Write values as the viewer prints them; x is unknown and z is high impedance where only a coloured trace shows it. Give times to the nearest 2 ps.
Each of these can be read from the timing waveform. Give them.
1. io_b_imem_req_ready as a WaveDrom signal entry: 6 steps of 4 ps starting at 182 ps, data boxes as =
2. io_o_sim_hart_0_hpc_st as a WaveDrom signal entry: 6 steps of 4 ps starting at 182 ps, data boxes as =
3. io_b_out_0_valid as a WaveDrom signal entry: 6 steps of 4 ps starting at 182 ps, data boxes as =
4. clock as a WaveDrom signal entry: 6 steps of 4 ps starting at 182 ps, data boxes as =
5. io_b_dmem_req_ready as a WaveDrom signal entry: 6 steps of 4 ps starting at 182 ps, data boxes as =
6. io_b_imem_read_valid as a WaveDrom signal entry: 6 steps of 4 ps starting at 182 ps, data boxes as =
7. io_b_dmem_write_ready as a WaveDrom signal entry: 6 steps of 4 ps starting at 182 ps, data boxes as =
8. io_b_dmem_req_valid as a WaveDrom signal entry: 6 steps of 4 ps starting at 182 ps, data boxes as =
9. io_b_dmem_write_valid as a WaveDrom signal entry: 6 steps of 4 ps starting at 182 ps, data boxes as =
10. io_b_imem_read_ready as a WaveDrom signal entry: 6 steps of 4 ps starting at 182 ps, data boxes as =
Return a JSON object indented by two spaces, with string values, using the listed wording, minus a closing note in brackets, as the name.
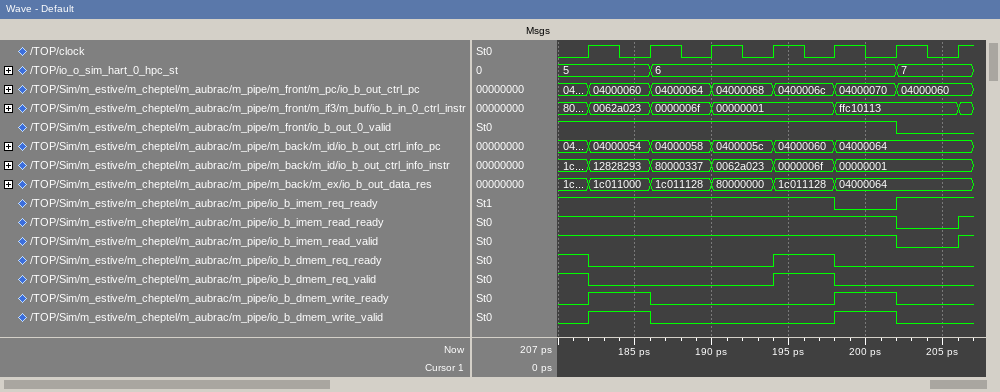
{
  "io_b_imem_req_ready as a WaveDrom signal entry: 6 steps of 4 ps starting at 182 ps, data boxes as =": "{name: 'io_b_imem_req_ready', wave: '1...01'}",
  "io_o_sim_hart_0_hpc_st as a WaveDrom signal entry: 6 steps of 4 ps starting at 182 ps, data boxes as =": "{name: 'io_o_sim_hart_0_hpc_st', wave: '==...=', data: '5 6 7'}",
  "io_b_out_0_valid as a WaveDrom signal entry: 6 steps of 4 ps starting at 182 ps, data boxes as =": "{name: 'io_b_out_0_valid', wave: '1....0'}",
  "clock as a WaveDrom signal entry: 6 steps of 4 ps starting at 182 ps, data boxes as =": "{name: 'clock', wave: 'p.....'}",
  "io_b_dmem_req_ready as a WaveDrom signal entry: 6 steps of 4 ps starting at 182 ps, data boxes as =": "{name: 'io_b_dmem_req_ready', wave: '0..10.'}",
  "io_b_imem_read_valid as a WaveDrom signal entry: 6 steps of 4 ps starting at 182 ps, data boxes as =": "{name: 'io_b_imem_read_valid', wave: '1....0'}",
  "io_b_dmem_write_ready as a WaveDrom signal entry: 6 steps of 4 ps starting at 182 ps, data boxes as =": "{name: 'io_b_dmem_write_ready', wave: '10..10'}",
  "io_b_dmem_req_valid as a WaveDrom signal entry: 6 steps of 4 ps starting at 182 ps, data boxes as =": "{name: 'io_b_dmem_req_valid', wave: '0..10.'}",
  "io_b_dmem_write_valid as a WaveDrom signal entry: 6 steps of 4 ps starting at 182 ps, data boxes as =": "{name: 'io_b_dmem_write_valid', wave: '10..10'}",
  "io_b_imem_read_ready as a WaveDrom signal entry: 6 steps of 4 ps starting at 182 ps, data boxes as =": "{name: 'io_b_imem_read_ready', wave: '1....0'}"
}
